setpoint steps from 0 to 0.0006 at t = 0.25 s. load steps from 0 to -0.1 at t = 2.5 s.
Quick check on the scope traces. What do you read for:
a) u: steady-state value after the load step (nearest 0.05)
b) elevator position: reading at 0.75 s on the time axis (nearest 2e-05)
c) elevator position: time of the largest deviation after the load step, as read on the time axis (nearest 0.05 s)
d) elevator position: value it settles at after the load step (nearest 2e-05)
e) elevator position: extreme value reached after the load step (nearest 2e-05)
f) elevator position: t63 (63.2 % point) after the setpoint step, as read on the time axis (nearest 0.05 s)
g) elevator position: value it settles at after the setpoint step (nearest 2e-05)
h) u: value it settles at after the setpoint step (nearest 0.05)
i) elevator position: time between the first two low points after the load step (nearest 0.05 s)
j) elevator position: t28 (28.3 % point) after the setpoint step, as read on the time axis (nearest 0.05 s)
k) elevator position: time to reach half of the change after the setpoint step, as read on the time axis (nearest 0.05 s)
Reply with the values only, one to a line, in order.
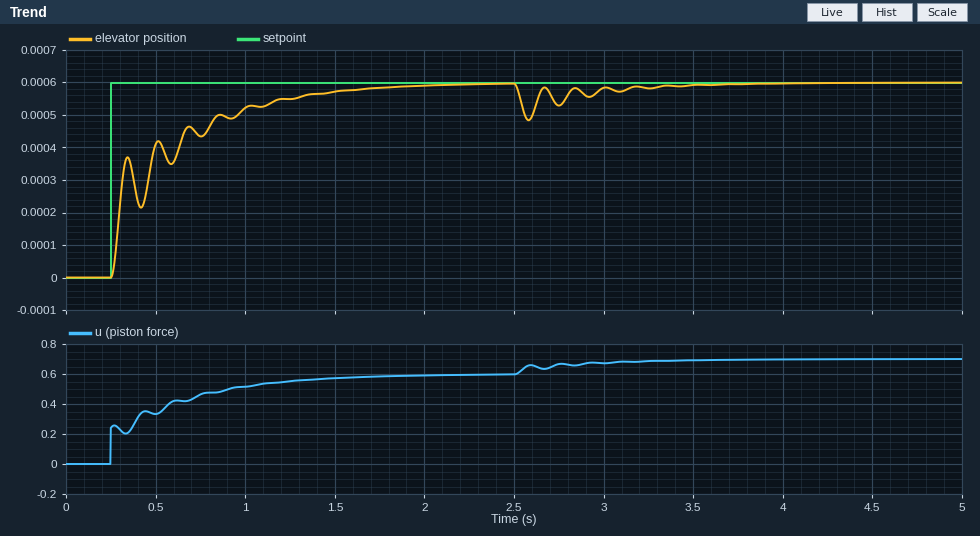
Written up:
0.70
0.00044
2.60 s
0.00060
0.00048
0.50 s
0.00060
0.60
0.15 s
0.30 s
0.30 s
